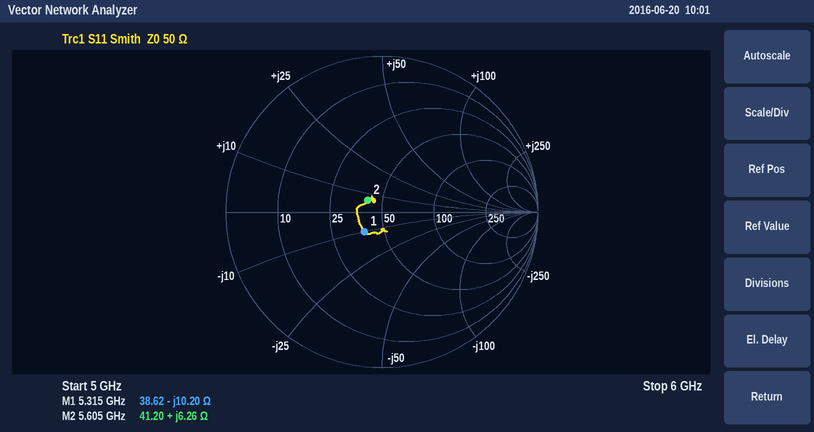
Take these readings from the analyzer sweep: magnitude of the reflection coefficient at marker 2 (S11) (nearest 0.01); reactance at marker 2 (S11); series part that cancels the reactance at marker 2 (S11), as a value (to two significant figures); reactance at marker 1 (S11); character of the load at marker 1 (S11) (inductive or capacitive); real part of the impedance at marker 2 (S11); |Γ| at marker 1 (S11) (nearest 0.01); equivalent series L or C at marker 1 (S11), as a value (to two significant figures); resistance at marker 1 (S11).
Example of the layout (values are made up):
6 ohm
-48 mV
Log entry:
0.12
+6.26 Ω
4.5 pF
-10.20 Ω
capacitive
41.20 Ω
0.17
2.9 pF
38.62 Ω
